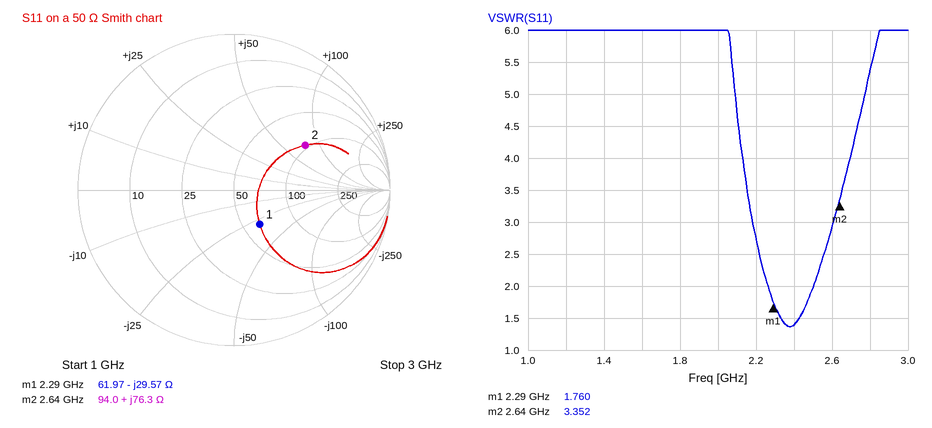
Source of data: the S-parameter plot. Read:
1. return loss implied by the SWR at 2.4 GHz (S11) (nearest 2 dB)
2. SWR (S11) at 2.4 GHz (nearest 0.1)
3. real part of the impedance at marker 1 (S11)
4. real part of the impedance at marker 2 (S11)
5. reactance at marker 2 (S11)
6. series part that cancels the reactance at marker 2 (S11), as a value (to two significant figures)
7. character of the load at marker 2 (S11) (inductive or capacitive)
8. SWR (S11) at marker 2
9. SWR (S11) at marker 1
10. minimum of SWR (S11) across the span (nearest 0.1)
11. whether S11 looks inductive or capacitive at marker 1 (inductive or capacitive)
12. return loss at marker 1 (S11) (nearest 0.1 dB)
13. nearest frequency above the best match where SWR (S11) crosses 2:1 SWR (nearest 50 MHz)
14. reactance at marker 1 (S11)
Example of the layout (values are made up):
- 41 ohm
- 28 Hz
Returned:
- 16 dB
- 1.4
- 61.97 Ω
- 94.0 Ω
- +76.3 Ω
- 790 fF
- inductive
- 3.352
- 1.760
- 1.4
- capacitive
- 11.2 dB
- 2.50 GHz
- -29.57 Ω
